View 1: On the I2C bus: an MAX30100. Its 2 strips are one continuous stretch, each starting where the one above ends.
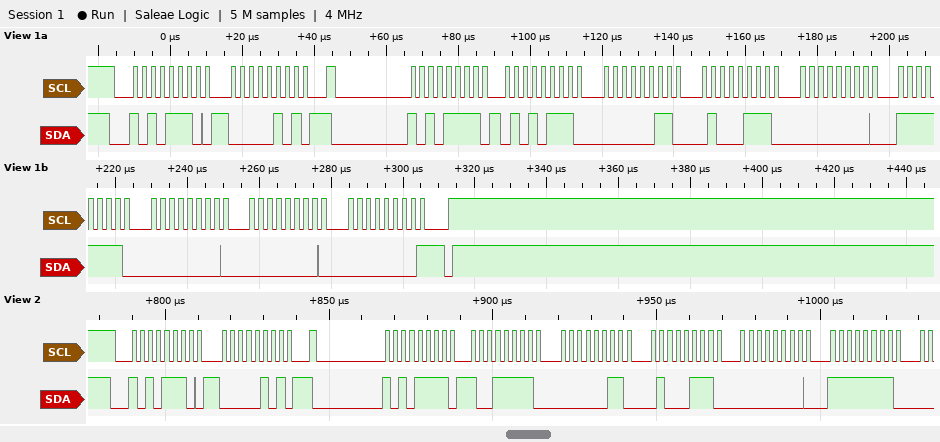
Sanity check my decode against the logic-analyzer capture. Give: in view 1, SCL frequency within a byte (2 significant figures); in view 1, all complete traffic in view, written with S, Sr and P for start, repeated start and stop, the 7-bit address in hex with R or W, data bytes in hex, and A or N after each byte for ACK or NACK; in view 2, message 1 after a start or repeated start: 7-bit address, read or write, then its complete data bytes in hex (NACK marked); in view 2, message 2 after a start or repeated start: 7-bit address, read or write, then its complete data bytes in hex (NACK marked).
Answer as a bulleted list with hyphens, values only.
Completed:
- 400 kHz
- S 57W A 05 A Sr 57R A 57 A 03 A 47 A 00 A FF A 00 A 00 A 00 N P
- 0x57 write: 05
- 0x57 read: 9F 03 47 00 FF
